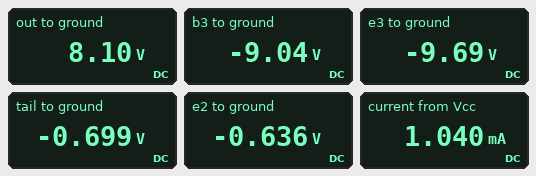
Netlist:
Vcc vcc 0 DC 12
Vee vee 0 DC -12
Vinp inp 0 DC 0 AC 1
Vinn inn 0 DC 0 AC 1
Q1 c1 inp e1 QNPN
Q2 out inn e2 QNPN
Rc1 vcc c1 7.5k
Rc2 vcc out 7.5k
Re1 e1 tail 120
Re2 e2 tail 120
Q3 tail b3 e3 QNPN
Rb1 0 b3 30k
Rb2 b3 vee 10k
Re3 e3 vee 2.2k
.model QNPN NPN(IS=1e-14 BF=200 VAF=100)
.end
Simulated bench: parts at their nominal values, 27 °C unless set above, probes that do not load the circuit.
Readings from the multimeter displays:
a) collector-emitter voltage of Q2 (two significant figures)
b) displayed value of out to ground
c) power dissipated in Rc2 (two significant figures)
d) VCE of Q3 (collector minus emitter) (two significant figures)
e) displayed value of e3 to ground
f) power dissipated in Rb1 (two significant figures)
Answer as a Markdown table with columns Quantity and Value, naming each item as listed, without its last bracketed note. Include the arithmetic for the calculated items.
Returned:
| Quantity | Value |
|---|---|
| collector-emitter voltage of Q2 | 8.1 V - (-636 mV) = 8.7 V |
| displayed value of out to ground | 8.10 V |
| power dissipated in Rc2 | (12 V - 8.1 V)^2 / 7.5 kΩ = 2.0 mW |
| VCE of Q3 (collector minus emitter) | -699 mV - (-9.69 V) = 9.0 V |
| displayed value of e3 to ground | -9.69 V |
| power dissipated in Rb1 | (0 V - (-9.04 V))^2 / 30 kΩ = 2.7 mW |
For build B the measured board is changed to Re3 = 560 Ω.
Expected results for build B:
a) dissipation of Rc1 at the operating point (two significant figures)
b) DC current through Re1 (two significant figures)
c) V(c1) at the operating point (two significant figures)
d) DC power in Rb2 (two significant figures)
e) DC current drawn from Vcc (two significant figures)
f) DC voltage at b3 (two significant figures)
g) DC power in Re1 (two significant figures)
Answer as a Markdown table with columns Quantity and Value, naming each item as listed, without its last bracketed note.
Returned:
| Quantity | Value |
|---|---|
| dissipation of Rc1 at the operating point | 21 mW |
| DC current through Re1 | 1.9 mA |
| V(c1) at the operating point | -620 mV |
| DC power in Rb2 | 820 µW |
| DC current drawn from Vcc | 3.4 mA |
| DC voltage at b3 | -9.1 V |
| DC power in Re1 | 450 µW |
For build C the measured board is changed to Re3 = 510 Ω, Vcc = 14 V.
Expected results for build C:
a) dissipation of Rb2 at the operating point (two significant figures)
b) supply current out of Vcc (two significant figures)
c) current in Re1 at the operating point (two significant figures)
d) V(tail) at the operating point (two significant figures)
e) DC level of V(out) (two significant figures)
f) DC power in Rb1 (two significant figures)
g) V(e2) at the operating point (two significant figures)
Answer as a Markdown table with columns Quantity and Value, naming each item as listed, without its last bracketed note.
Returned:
| Quantity | Value |
|---|---|
| dissipation of Rb2 at the operating point | 810 µW |
| supply current out of Vcc | 3.9 mA |
| current in Re1 at the operating point | 2.1 mA |
| V(tail) at the operating point | -930 mV |
| DC level of V(out) | -610 mV |
| DC power in Rb1 | 2.8 mW |
| V(e2) at the operating point | -680 mV |
